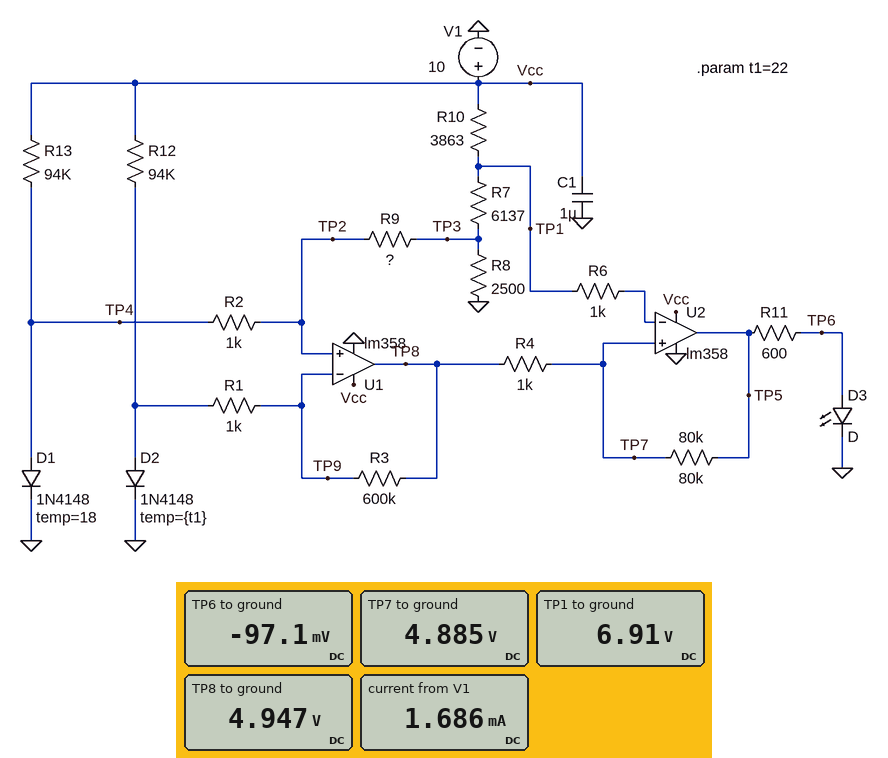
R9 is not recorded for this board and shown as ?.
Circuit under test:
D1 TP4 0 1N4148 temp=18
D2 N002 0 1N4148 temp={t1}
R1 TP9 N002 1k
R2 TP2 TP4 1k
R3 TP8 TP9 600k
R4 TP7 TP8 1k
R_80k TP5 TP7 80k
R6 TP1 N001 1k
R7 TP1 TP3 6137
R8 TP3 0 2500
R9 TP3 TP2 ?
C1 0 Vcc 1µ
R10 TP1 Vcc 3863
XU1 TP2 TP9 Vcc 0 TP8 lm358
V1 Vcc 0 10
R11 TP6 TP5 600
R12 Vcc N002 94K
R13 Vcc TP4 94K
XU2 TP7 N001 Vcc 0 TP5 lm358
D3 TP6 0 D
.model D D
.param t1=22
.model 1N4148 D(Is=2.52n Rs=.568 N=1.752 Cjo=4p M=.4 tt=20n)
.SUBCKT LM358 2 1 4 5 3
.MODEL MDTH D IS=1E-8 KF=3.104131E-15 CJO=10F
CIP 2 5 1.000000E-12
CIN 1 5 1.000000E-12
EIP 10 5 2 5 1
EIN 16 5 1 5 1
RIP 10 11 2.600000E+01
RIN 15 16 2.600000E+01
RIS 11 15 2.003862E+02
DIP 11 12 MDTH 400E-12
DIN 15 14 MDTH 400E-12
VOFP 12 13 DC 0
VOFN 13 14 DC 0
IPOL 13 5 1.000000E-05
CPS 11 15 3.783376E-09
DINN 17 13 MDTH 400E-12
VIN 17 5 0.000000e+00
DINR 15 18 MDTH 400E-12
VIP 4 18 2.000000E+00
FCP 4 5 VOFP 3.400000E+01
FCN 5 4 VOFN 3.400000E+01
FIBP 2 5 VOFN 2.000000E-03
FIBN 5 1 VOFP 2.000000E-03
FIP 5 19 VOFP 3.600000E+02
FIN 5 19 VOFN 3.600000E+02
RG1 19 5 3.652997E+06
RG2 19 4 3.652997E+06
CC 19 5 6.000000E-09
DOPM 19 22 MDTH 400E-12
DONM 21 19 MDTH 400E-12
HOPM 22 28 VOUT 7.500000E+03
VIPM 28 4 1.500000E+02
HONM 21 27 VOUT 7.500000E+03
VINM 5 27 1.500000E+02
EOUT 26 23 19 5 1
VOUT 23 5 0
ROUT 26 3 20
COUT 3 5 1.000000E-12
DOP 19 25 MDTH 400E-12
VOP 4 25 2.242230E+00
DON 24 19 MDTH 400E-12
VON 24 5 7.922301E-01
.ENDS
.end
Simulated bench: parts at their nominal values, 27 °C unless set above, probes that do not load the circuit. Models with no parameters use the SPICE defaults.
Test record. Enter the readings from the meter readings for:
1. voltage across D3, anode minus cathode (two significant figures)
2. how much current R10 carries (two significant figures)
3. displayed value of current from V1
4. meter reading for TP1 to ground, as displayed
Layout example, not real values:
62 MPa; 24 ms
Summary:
-97 mV; 800 µA; 1.686 mA; 6.91 V
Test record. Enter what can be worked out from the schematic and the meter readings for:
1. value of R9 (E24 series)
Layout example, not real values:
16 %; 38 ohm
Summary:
1.8 MΩ
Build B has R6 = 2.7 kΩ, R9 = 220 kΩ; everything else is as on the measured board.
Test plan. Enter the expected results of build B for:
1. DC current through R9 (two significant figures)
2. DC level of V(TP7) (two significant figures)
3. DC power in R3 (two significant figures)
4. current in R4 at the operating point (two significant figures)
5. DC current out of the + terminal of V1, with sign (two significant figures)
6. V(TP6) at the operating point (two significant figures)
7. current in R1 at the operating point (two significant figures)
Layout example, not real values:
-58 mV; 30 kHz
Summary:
6.7 µA; 8.5 V; 110 µW; 1.0 µA; -1.9 mA; 720 mV; 13 µA
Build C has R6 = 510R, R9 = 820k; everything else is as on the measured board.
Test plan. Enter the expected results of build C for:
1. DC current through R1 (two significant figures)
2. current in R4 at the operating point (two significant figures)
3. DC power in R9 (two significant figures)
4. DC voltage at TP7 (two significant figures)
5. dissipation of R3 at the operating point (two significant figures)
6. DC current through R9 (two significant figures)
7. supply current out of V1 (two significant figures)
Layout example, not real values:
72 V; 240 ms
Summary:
8.4 µA; 70 µA; 2.7 µW; 5.5 V; 42 µW; 1.8 µA; 1.7 mA
